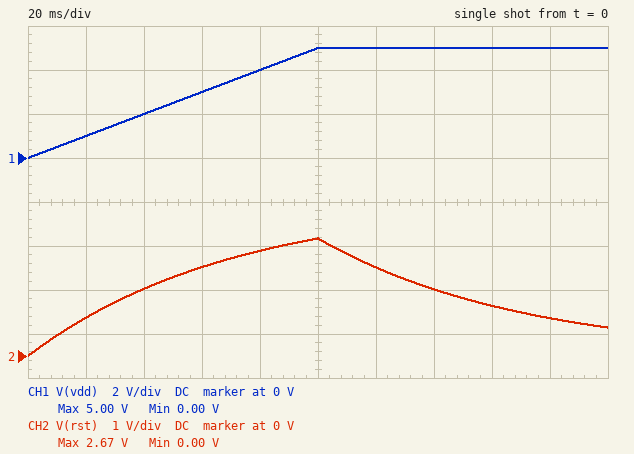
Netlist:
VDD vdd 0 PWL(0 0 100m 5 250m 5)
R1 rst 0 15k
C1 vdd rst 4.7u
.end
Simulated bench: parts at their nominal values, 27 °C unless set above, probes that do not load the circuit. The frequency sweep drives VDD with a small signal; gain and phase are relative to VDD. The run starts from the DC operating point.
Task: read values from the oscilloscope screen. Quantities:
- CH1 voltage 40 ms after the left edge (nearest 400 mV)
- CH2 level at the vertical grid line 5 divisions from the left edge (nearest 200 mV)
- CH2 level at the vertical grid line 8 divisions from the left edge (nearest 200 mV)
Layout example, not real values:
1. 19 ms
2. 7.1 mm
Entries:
1. 2.0 V
2. 2.6 V
3. 1.2 V
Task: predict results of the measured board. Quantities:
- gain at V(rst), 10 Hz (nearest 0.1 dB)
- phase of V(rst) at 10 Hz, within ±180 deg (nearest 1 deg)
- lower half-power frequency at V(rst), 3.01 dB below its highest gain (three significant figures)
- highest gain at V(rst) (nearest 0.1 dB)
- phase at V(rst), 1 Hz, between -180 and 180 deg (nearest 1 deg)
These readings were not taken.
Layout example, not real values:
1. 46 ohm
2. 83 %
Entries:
1. -0.2 dB
2. 13 deg
3. 2.26 Hz
4. 0 dB
5. 66 deg
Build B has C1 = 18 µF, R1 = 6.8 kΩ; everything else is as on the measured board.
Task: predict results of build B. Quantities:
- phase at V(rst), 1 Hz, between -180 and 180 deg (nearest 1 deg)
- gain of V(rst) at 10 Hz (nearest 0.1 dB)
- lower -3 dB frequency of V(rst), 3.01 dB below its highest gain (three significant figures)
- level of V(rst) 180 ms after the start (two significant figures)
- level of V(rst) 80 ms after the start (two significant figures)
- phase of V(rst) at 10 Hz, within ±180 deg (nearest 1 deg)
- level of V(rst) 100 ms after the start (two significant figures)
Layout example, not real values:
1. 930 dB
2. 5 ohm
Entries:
1. 52 deg
2. -0.1 dB
3. 1.30 Hz
4. 1.8 V
5. 2.9 V
6. 7 deg
7. 3.4 V
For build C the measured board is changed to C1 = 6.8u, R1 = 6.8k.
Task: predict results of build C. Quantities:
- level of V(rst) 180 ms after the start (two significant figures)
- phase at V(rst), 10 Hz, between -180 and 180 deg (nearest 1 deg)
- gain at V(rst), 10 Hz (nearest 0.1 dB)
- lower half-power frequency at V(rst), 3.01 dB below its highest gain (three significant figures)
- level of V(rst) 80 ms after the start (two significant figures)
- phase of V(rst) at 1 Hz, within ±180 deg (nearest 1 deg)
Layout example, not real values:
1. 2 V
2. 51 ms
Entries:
1. 360 mV
2. 19 deg
3. -0.5 dB
4. 3.44 Hz
5. 1.9 V
6. 74 deg
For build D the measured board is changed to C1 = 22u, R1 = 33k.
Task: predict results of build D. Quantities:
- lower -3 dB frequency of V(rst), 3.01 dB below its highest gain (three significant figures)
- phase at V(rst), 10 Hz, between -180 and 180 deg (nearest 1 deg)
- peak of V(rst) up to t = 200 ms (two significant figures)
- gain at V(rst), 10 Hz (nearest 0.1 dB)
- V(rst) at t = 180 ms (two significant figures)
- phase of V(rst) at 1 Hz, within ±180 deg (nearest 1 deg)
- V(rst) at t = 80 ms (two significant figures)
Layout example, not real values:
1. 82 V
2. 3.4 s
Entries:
1. 219 mHz
2. 1 deg
3. 4.7 V
4. 0 dB
5. 4.2 V
6. 12 deg
7. 3.8 V
